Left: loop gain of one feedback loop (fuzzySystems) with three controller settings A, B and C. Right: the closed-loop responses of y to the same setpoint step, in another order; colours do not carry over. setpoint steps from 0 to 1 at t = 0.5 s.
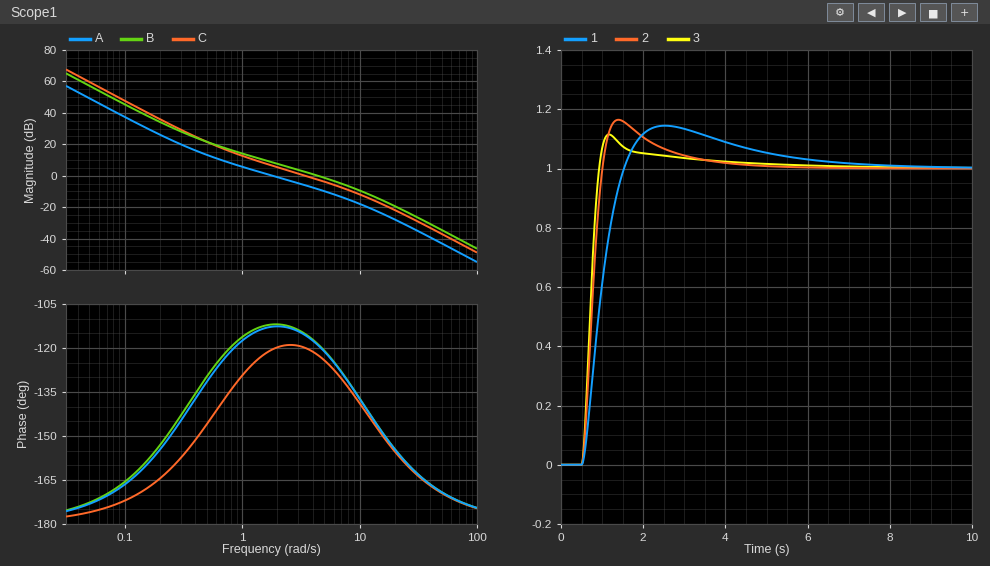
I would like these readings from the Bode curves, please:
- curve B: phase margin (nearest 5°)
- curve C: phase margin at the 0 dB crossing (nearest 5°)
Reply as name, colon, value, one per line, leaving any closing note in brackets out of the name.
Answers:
curve B: phase margin: 60°
curve C: phase margin at the 0 dB crossing: 60°
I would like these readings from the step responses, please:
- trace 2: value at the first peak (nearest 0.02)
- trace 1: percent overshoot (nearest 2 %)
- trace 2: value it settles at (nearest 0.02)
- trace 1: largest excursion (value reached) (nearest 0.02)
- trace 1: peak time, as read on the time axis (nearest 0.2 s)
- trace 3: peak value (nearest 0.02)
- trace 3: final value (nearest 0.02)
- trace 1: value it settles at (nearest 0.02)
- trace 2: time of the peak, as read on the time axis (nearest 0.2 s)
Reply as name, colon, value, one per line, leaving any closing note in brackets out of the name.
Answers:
trace 2: value at the first peak: 1.16
trace 1: percent overshoot: 14 %
trace 2: value it settles at: 1.00
trace 1: largest excursion (value reached): 1.14
trace 1: peak time, as read on the time axis: 2.6 s
trace 3: peak value: 1.12
trace 3: final value: 1.00
trace 1: value it settles at: 1.00
trace 2: time of the peak, as read on the time axis: 1.4 s
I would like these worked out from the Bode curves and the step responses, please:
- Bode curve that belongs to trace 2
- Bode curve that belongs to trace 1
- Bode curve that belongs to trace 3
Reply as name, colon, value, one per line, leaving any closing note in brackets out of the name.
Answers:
Bode curve that belongs to trace 2: C
Bode curve that belongs to trace 1: A
Bode curve that belongs to trace 3: B
